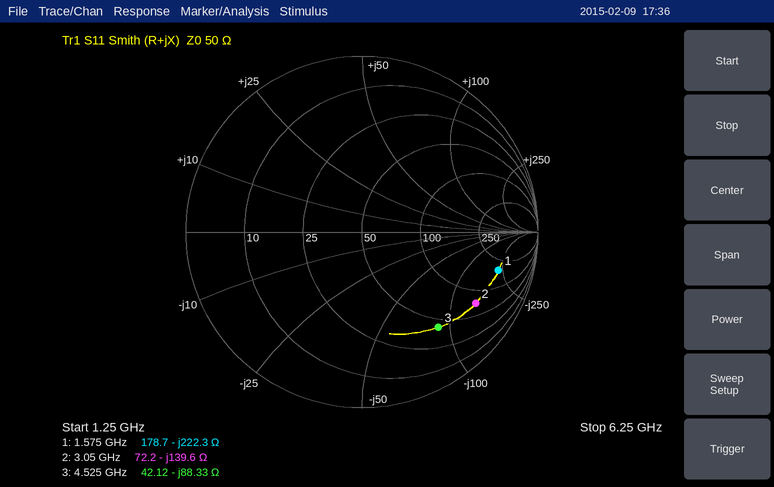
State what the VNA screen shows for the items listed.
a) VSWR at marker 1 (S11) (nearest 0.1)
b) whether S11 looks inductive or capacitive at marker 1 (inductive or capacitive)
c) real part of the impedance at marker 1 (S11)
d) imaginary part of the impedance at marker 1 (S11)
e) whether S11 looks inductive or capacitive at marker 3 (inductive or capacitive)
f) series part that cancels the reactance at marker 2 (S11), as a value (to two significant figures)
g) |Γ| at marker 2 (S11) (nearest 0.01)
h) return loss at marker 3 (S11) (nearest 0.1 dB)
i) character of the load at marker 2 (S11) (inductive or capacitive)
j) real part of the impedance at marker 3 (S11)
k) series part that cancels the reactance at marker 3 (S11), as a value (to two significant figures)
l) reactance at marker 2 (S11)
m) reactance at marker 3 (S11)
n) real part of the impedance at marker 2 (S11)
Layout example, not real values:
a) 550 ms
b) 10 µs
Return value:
a) 9.3
b) capacitive
c) 178.7 Ω
d) -222.3 Ω
e) capacitive
f) 7.3 nH
g) 0.76
h) 3.2 dB
i) capacitive
j) 42.12 Ω
k) 3.1 nH
l) -139.6 Ω
m) -88.33 Ω
n) 72.2 Ω
